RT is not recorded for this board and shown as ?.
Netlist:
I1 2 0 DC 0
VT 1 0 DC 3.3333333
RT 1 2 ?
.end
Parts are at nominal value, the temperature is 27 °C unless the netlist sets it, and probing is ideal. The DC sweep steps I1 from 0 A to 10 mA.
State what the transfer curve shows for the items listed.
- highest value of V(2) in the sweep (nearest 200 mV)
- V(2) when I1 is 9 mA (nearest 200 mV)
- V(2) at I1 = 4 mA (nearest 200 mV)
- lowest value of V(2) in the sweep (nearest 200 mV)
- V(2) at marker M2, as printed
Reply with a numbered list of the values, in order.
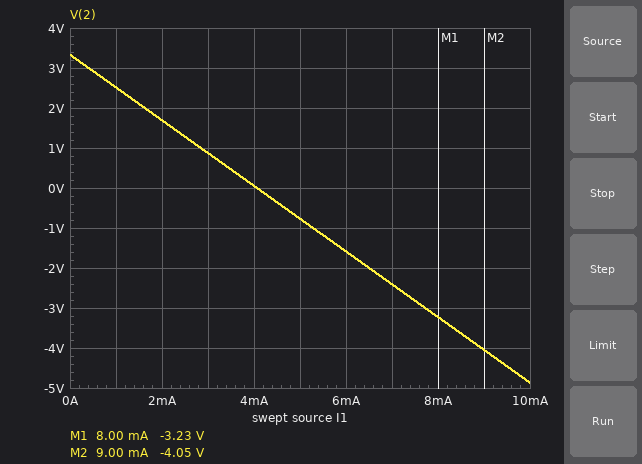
1. 3.4 V
2. -4.0 V
3. 0 V
4. -4.8 V
5. -4.05 V
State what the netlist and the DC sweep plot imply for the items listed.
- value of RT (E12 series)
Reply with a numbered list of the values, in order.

1. 820 Ω
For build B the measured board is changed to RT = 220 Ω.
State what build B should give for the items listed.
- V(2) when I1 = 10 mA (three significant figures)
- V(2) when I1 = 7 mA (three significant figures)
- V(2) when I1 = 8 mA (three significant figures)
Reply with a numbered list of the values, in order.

1. 1.13 V
2. 1.79 V
3. 1.57 V
